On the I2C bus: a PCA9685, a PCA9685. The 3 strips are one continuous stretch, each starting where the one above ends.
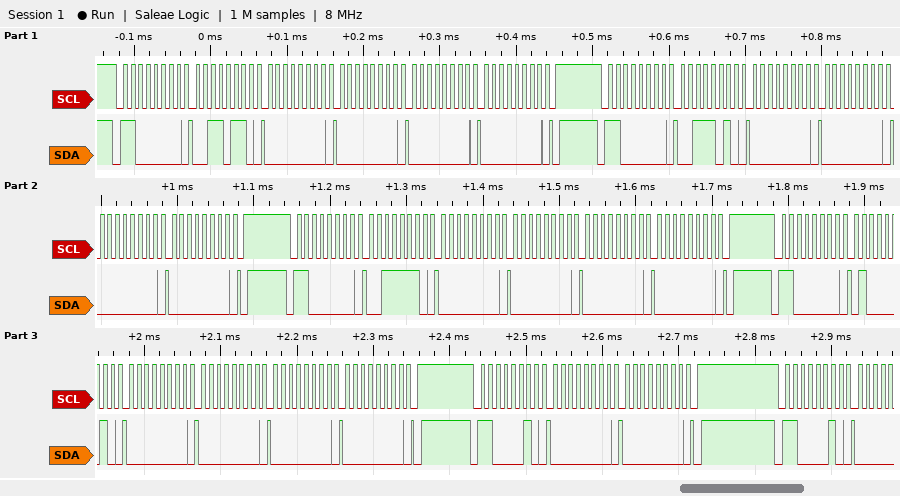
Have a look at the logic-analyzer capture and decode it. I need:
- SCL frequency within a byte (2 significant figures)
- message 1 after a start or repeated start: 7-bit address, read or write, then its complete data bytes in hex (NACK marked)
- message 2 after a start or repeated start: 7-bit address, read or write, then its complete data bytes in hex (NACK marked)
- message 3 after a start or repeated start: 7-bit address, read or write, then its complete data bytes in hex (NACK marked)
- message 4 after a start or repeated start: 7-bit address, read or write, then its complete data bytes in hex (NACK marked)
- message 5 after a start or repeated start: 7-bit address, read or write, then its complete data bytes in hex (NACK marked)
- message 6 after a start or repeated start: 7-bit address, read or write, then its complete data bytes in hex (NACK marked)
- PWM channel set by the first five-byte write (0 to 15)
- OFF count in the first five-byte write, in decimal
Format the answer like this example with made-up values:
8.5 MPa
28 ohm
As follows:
100 kHz
0x60 write: 36 00 00 00 00
0x60 write: 3A 00 00 00 00
0x60 write: 3E 00 00 00 00
0x60 write: 42 00 00 00 00
0x61 write: 00 00
0x61 write
12
0
